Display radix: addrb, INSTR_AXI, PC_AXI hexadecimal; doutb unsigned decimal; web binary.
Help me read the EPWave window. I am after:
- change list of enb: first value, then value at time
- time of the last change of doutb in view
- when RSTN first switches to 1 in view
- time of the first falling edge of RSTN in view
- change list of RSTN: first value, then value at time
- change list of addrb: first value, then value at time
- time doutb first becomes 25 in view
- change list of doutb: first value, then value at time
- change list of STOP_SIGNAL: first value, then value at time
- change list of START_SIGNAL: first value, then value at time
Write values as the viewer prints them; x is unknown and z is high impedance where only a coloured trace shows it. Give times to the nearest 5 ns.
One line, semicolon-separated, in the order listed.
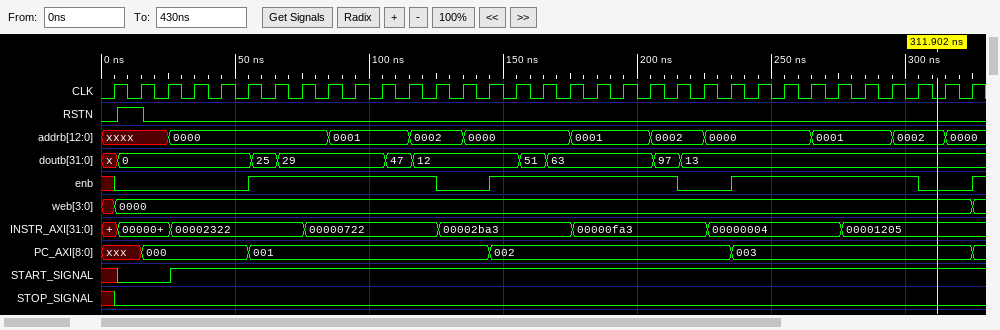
x, 0 at 5 ns, 1 at 55 ns, 0 at 125 ns, 1 at 145 ns, 0 at 215 ns, 1 at 235 ns, 0 at 305 ns, 1 at 325 ns; 215 ns; 5 ns; 15 ns; 0, 1 at 5 ns, 0 at 15 ns; xxxx, 0000 at 25 ns, 0001 at 85 ns, 0002 at 115 ns, 0000 at 135 ns, 0001 at 175 ns, 0002 at 205 ns, 0000 at 225 ns, 0001 at 265 ns, 0002 at 295 ns, 0000 at 315 ns; 55 ns; x, 0 at 5 ns, 25 at 55 ns, 29 at 65 ns, 47 at 105 ns, 12 at 115 ns, 51 at 155 ns, 63 at 165 ns, 97 at 205 ns, 13 at 215 ns; x, 0 at 5 ns; x, 0 at 5 ns, 1 at 25 ns
